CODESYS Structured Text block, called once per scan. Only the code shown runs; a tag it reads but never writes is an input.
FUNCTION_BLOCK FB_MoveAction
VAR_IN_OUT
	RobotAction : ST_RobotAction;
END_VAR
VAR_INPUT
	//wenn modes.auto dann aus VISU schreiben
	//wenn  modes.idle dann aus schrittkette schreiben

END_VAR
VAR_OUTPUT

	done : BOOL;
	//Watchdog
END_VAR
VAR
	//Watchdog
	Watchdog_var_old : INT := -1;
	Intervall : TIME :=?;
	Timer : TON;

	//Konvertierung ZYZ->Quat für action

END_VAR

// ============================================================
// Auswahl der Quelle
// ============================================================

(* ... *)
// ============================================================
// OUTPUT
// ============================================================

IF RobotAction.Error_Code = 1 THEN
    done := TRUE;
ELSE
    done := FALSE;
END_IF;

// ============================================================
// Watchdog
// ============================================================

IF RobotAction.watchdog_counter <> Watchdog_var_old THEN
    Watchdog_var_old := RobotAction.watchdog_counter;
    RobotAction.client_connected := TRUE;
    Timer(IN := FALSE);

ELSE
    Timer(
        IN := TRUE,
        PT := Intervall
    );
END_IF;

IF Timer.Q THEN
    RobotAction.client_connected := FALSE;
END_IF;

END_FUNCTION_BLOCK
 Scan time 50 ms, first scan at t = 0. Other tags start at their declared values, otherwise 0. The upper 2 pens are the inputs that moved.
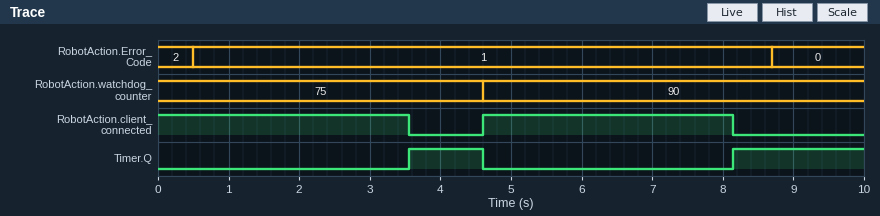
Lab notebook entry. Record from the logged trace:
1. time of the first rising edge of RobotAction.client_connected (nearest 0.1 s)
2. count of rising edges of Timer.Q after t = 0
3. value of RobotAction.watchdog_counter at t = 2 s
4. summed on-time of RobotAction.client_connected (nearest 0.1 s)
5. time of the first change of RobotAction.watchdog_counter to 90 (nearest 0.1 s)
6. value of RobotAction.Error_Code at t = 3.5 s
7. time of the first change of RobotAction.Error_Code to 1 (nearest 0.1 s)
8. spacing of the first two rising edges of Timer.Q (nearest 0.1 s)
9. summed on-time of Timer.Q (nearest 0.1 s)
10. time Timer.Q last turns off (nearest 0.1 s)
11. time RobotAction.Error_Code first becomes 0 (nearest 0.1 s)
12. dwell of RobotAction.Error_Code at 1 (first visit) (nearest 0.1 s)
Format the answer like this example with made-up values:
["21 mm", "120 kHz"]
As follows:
["4.6 s", "2", "75", "7.1 s", "4.6 s", "1", "0.5 s", "4.6 s", "2.9 s", "4.6 s", "8.7 s", "8.2 s"]
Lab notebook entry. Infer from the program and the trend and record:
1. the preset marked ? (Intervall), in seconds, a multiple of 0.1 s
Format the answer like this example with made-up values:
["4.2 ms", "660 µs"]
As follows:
["3.5 s"]
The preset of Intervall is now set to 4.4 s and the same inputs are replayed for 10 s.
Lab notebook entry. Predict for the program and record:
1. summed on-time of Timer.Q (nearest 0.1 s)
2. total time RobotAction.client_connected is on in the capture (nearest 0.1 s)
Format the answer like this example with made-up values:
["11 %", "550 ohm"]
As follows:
["1.1 s", "8.9 s"]
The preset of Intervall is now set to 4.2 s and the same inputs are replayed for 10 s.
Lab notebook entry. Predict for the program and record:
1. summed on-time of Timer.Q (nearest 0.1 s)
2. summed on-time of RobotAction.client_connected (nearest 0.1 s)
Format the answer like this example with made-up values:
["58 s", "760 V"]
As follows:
["1.5 s", "8.5 s"]
